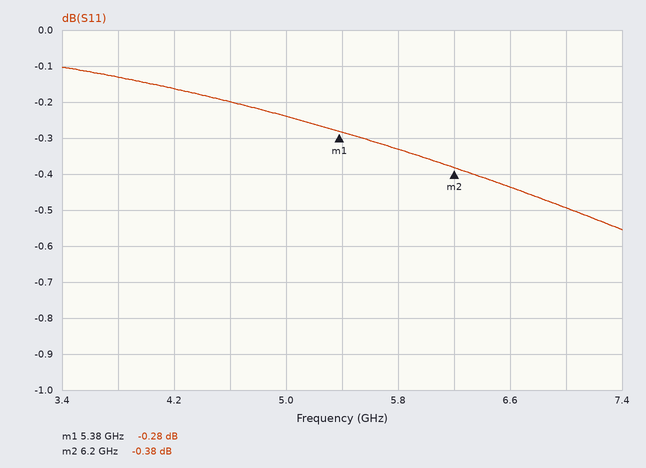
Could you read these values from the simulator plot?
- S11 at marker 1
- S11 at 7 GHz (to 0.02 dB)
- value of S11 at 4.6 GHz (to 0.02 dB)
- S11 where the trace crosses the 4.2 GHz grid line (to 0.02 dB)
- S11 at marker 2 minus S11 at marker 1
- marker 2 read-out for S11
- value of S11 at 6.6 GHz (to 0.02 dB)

-0.28 dB
-0.50 dB
-0.20 dB
-0.16 dB
-0.10 dB
-0.38 dB
-0.44 dB
